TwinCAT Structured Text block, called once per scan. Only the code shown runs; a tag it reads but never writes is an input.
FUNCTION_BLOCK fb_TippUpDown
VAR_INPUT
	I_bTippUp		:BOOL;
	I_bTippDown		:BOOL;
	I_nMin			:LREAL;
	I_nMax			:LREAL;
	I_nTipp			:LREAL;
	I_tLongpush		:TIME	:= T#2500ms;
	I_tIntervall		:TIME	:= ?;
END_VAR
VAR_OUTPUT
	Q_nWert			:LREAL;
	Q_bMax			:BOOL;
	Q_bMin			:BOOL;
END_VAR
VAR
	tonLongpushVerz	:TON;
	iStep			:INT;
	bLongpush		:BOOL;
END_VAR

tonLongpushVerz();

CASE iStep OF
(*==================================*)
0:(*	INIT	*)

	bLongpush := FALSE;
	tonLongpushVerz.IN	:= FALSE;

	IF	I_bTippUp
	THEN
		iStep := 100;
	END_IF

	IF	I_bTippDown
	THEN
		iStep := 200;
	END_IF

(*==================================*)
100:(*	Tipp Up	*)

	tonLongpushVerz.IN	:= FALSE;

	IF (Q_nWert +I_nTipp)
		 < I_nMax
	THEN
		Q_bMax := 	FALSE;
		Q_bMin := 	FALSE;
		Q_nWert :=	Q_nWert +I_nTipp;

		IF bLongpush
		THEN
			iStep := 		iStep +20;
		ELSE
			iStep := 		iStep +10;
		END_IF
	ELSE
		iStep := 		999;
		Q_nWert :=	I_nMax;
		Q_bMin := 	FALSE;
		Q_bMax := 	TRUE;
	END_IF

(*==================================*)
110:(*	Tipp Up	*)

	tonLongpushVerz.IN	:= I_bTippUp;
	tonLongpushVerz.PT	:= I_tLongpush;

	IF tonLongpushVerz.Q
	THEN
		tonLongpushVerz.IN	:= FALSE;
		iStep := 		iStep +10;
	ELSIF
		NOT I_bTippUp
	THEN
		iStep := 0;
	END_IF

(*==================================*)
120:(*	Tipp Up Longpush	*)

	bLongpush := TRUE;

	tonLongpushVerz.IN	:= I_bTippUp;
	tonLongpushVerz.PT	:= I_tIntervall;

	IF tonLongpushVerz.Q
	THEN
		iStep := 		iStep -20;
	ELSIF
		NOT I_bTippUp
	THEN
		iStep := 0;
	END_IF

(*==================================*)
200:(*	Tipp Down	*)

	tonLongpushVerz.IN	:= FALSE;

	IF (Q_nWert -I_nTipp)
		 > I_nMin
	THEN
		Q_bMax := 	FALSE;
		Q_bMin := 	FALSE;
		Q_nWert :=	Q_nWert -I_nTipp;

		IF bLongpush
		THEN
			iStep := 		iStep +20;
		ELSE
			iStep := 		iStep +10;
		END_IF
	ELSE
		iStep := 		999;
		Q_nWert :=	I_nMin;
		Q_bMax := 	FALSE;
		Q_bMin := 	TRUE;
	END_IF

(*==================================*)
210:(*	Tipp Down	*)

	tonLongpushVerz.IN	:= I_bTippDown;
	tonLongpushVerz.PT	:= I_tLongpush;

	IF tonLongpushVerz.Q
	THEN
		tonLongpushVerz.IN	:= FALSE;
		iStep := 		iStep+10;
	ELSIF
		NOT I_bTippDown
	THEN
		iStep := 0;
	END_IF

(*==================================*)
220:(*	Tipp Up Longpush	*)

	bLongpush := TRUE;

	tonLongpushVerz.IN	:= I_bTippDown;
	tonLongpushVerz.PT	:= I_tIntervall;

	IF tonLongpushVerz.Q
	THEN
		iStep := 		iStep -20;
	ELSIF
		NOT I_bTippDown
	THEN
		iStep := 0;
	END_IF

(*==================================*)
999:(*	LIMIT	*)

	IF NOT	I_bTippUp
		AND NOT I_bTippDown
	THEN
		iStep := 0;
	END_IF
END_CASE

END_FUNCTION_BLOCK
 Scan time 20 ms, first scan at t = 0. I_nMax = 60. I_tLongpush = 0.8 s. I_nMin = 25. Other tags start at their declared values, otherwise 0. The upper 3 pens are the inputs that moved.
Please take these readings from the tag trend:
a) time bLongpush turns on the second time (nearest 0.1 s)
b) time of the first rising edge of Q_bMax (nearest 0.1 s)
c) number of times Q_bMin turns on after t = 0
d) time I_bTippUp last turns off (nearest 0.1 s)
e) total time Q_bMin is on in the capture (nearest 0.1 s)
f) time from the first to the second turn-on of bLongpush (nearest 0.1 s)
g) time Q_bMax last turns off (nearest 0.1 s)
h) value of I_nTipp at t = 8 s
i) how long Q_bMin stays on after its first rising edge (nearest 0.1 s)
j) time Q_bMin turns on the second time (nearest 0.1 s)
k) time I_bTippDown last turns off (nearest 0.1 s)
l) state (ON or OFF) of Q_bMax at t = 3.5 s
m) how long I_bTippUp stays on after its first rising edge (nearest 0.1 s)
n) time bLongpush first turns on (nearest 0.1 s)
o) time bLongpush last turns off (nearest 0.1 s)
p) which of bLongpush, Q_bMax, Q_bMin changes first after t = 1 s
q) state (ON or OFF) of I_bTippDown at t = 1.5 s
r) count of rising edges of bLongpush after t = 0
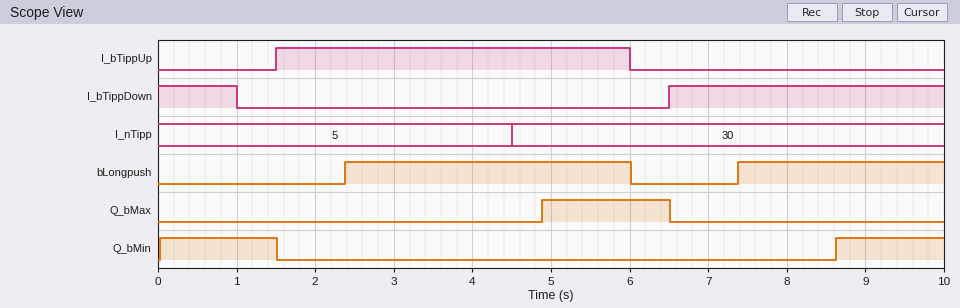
7.4 s
4.9 s
2
6.0 s
2.9 s
5.0 s
6.5 s
30
1.5 s
8.6 s
1.0 s
OFF
4.5 s
2.4 s
6.0 s
Q_bMin
OFF
2
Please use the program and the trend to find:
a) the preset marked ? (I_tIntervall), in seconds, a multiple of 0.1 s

1.2 s
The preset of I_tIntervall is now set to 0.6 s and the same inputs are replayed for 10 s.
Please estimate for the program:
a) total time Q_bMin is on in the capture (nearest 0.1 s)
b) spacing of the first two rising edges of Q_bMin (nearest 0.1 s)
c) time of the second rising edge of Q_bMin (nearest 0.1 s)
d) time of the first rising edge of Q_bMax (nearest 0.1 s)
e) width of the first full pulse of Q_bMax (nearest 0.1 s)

3.5 s
8.0 s
8.0 s
5.0 s
1.5 s
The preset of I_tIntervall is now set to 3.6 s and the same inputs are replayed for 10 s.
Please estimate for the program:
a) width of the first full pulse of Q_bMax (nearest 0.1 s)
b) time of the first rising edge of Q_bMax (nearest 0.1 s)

0.5 s
6.0 s
